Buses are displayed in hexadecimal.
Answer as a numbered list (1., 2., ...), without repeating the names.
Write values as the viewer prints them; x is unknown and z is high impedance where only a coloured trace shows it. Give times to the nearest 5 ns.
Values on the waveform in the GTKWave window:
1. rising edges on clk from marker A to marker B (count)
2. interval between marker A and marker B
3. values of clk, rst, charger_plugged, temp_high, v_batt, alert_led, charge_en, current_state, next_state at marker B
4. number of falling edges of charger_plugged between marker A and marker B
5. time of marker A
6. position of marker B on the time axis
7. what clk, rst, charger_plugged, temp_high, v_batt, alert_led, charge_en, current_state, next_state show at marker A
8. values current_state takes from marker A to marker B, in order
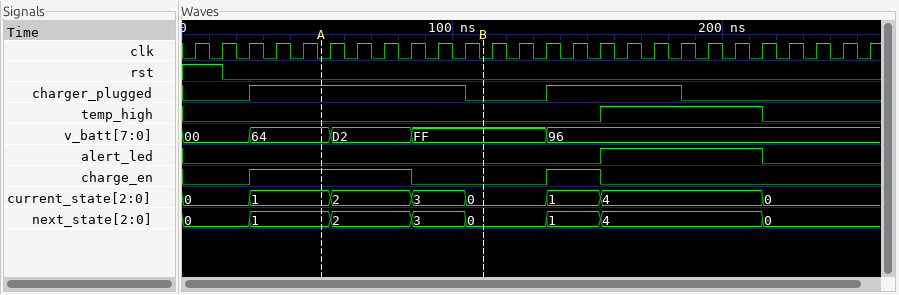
1. 6
2. 60 ns
3. clk=0, rst=0, charger_plugged=0, temp_high=0, v_batt=FF, alert_led=0, charge_en=0, current_state=0, next_state=0
4. 1
5. 50 ns
6. 110 ns
7. clk=0, rst=0, charger_plugged=1, temp_high=0, v_batt=64, alert_led=0, charge_en=1, current_state=1, next_state=1
8. 1, 2, 3, 0
